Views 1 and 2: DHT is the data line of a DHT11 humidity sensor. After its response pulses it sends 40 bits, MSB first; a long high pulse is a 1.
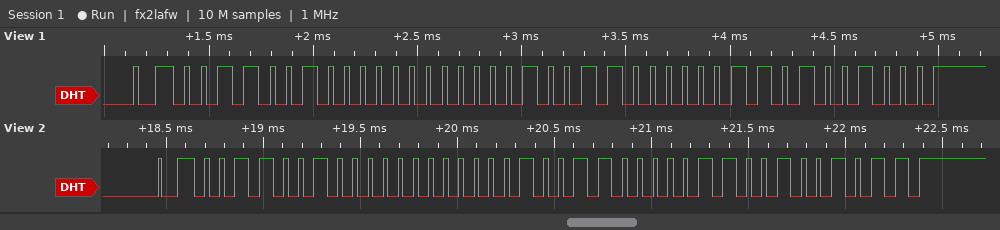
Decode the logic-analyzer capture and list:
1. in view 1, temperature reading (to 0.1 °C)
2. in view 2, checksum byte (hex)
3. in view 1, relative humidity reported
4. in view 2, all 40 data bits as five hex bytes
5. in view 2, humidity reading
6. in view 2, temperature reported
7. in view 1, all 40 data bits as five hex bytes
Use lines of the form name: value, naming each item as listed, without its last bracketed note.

in view 1, temperature reading: 19.3 °C
in view 2, checksum byte: 0x4B
in view 1, relative humidity reported: 50 %
in view 2, all 40 data bits as five hex bytes: 32 00 13 06 4B
in view 2, humidity reading: 50 %
in view 2, temperature reported: 19.6 °C
in view 1, all 40 data bits as five hex bytes: 32 00 13 03 48
